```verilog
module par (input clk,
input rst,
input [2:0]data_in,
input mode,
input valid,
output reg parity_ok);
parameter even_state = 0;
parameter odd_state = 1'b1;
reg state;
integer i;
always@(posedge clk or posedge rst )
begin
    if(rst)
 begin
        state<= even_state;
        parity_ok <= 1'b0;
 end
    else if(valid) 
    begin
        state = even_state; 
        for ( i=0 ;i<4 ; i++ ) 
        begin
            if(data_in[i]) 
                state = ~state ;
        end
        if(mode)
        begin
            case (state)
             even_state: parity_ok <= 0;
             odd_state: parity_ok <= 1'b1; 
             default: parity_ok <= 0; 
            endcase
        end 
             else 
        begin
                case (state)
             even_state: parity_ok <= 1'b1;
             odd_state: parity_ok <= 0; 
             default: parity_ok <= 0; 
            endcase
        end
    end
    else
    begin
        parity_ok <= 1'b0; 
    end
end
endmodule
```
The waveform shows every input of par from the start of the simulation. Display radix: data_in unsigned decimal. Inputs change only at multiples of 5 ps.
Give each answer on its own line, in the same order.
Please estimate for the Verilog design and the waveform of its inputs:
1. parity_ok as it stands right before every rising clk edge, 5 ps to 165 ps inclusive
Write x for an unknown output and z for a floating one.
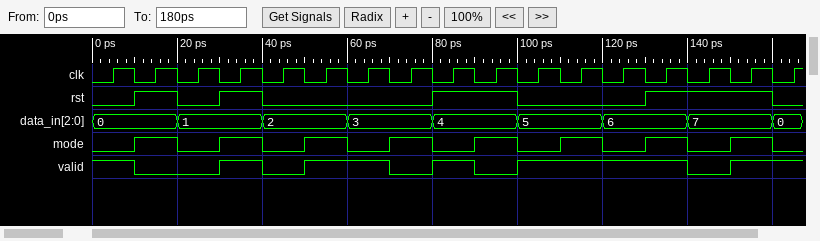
x 0 0 0 0 0 1 1 0 0 0 1 0 0 0 0 0
